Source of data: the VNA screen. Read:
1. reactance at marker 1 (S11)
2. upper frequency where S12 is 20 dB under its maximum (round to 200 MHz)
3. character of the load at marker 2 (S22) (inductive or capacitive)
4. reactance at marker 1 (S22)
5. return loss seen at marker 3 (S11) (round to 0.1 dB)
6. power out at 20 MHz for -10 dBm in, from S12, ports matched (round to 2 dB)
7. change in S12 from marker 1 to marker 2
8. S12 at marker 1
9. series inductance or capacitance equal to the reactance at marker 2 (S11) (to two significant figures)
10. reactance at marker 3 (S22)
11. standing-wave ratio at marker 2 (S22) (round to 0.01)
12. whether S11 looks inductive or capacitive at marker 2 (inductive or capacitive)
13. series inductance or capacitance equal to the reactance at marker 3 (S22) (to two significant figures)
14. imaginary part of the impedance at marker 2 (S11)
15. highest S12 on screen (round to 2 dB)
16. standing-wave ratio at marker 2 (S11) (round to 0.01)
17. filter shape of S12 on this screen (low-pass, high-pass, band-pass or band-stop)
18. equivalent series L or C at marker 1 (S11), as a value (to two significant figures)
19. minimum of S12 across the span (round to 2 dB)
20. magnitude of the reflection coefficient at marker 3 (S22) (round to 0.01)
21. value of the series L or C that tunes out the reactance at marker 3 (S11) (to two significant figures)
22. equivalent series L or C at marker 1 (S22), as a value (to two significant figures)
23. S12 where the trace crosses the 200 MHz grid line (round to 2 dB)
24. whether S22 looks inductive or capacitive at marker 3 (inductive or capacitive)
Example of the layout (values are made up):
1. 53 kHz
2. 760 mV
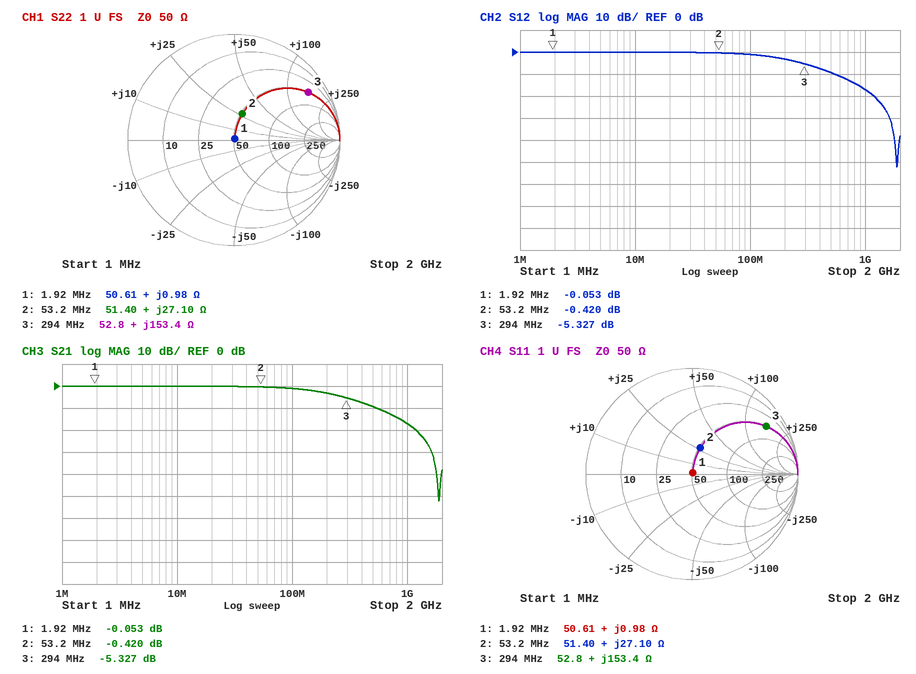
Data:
1. +0.98 Ω
2. 1.2 GHz
3. inductive
4. +0.98 Ω
5. 1.6 dB
6. -10 dBm
7. -0.367 dB
8. -0.053 dB
9. 81 nH
10. +153.4 Ω
11. 1.70
12. inductive
13. 83 nH
14. +27.10 Ω
15. 0 dB
16. 1.70
17. low-pass
18. 81 nH
19. -52 dB
20. 0.83
21. 3.5 pF
22. 81 nH
23. -4 dB
24. inductive
